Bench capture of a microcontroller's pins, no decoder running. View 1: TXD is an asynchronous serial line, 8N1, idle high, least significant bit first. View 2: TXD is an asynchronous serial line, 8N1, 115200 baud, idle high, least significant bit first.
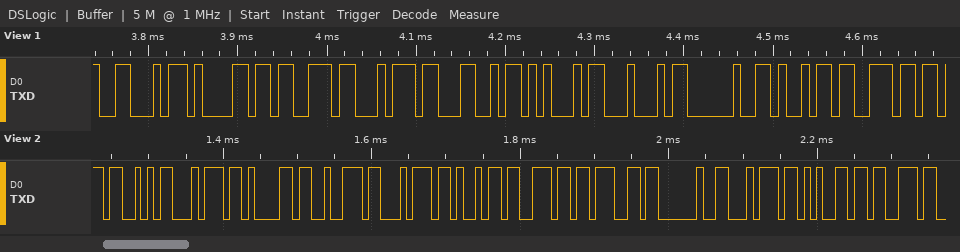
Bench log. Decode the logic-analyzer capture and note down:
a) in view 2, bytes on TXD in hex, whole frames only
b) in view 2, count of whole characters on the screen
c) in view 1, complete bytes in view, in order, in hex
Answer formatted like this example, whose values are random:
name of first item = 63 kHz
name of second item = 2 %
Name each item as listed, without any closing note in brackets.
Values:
in view 2, bytes on TXD in hex, whole frames only = 53 74 61 72 74 69 6E 67 20 74 65 73
in view 2, count of whole characters on the screen = 12
in view 1, complete bytes in view, in order, in hex = 0x46 0x61 0x73 0x74 0x4C 0x45 0x44 0x20 0x69 0x6E
